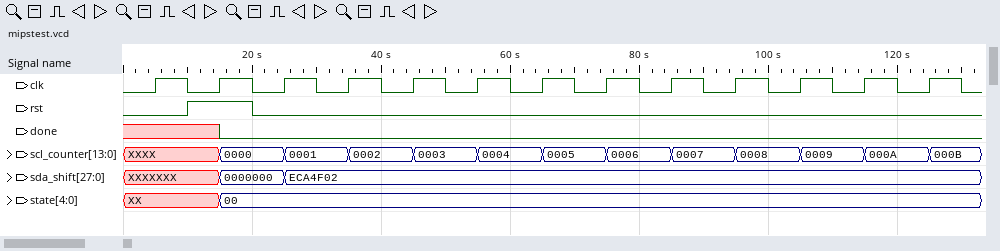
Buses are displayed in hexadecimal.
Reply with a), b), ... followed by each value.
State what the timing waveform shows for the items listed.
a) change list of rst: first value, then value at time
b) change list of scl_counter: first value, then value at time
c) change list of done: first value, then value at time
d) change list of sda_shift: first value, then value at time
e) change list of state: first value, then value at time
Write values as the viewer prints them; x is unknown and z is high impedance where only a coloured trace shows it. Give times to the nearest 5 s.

a) 0, 1 at 10 s, 0 at 20 s
b) XXXX, 0000 at 15 s, 0001 at 25 s, 0002 at 35 s, 0003 at 45 s, 0004 at 55 s, 0005 at 65 s, 0006 at 75 s, 0007 at 85 s, 0008 at 95 s, 0009 at 105 s, 000A at 115 s, 000B at 125 s
c) x, 0 at 15 s
d) XXXXXXX, 0000000 at 15 s, ECA4F02 at 25 s
e) XX, 00 at 15 s
